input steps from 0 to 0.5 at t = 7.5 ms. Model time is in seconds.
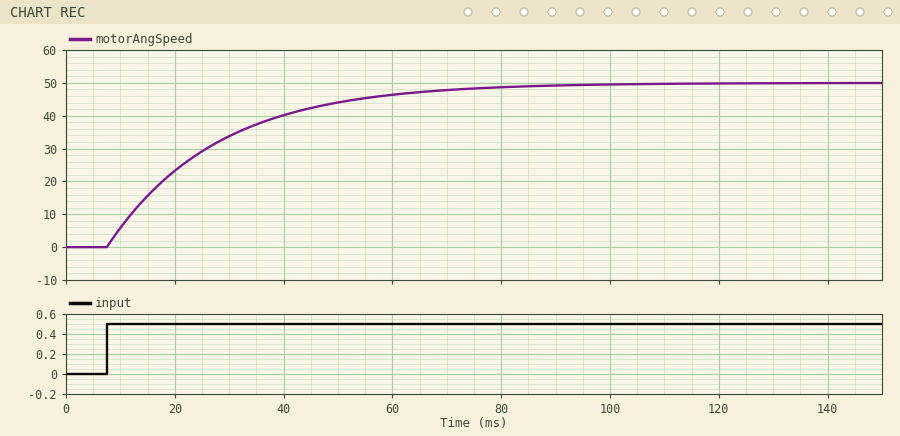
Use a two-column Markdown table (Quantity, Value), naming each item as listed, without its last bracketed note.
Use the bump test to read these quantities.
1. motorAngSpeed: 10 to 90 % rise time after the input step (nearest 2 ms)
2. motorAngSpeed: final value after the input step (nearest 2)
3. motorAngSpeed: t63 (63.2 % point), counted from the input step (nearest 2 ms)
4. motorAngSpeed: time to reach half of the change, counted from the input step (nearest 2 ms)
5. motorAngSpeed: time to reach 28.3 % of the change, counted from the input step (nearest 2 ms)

| Quantity | Value |
|---|---|
| motorAngSpeed: 10 to 90 % rise time after the input step | 44 ms |
| motorAngSpeed: final value after the input step | 50 |
| motorAngSpeed: t63 (63.2 % point), counted from the input step | 20 ms |
| motorAngSpeed: time to reach half of the change, counted from the input step | 14 ms |
| motorAngSpeed: time to reach 28.3 % of the change, counted from the input step | 6 ms |
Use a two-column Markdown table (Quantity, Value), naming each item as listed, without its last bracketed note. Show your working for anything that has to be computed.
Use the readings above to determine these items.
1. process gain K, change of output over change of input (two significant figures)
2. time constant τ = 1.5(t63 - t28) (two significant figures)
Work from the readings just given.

| Quantity | Value |
|---|---|
| process gain K, change of output over change of input | (50 - 0) / 0.5 = 100 |
| time constant τ = 1.5(t63 - t28) | 1.5 × (20 - 6) = 21 ms |
